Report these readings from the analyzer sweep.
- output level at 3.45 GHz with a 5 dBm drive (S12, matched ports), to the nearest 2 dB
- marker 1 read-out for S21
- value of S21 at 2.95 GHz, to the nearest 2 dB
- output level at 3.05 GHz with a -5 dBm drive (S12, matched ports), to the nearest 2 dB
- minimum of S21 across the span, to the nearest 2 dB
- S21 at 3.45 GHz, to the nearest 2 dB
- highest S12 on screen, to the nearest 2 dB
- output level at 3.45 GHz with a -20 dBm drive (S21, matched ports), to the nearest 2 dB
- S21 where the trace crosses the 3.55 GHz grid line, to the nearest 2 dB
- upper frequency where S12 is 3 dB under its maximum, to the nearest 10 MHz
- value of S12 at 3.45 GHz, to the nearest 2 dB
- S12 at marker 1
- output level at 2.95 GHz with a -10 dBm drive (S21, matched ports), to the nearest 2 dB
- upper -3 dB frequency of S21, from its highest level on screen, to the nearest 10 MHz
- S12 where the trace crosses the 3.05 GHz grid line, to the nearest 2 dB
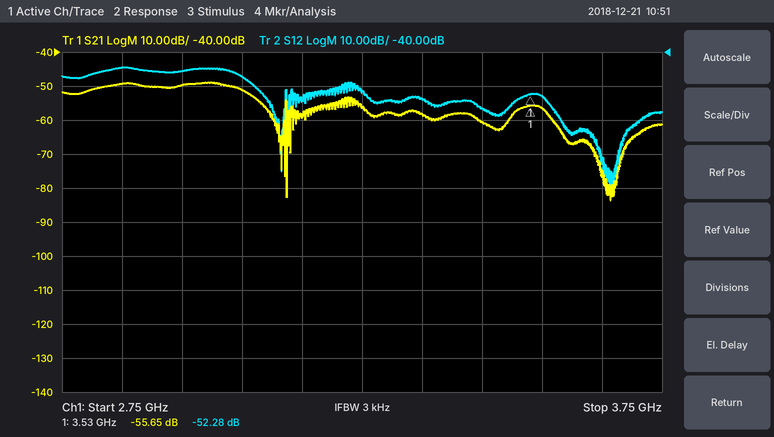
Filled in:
-52 dBm
-55.65 dB
-50 dB
-52 dBm
-84 dB
-60 dB
-44 dB
-80 dBm
-56 dB
3.05 GHz
-56 dB
-52.28 dB
-60 dBm
3.06 GHz
-48 dB
